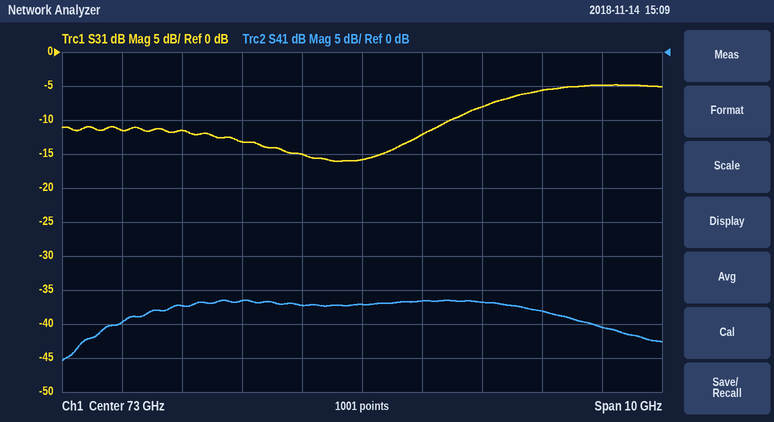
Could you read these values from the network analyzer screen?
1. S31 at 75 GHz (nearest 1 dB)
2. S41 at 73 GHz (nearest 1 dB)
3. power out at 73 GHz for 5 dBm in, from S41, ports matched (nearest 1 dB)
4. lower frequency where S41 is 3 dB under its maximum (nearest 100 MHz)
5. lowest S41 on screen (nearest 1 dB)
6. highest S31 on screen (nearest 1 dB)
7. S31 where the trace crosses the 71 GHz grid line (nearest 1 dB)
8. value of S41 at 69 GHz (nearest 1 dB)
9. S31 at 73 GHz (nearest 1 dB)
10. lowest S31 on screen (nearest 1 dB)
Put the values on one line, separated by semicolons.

-8 dB; -37 dB; -32 dBm; 69.0 GHz; -45 dB; -5 dB; -13 dB; -40 dB; -16 dB; -16 dB
